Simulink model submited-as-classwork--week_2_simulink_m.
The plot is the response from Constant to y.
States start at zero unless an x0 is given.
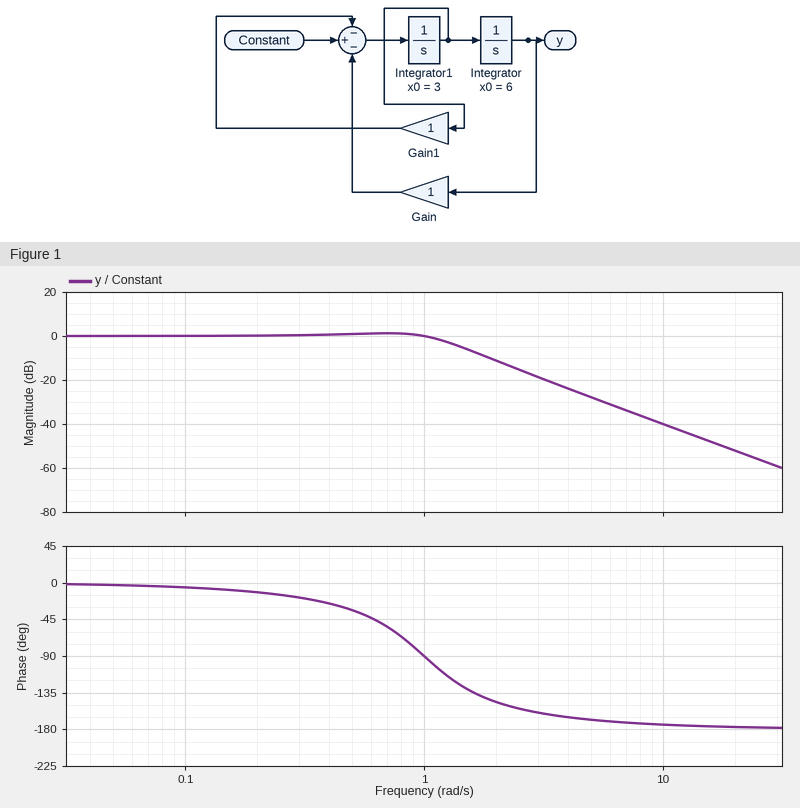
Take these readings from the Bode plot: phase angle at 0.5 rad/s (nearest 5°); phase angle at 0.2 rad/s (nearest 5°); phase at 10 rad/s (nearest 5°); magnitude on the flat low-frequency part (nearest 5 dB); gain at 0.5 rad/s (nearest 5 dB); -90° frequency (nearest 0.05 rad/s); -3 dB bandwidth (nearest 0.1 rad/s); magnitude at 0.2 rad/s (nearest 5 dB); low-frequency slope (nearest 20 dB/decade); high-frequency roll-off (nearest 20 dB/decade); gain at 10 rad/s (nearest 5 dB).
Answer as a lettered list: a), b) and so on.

a) -35°
b) -10°
c) -175°
d) 0 dB
e) 0 dB
f) 1.00 rad/s
g) 1.3 rad/s
h) 0 dB
i) 0 dB/decade
j) -40 dB/decade
k) -40 dB
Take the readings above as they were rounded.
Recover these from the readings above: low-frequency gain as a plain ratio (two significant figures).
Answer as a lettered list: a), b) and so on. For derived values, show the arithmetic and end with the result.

a) 10^(0 / 20) = 1.0
